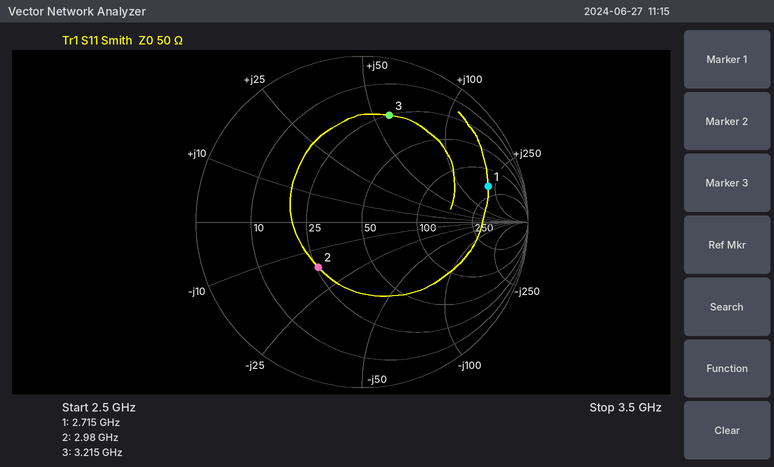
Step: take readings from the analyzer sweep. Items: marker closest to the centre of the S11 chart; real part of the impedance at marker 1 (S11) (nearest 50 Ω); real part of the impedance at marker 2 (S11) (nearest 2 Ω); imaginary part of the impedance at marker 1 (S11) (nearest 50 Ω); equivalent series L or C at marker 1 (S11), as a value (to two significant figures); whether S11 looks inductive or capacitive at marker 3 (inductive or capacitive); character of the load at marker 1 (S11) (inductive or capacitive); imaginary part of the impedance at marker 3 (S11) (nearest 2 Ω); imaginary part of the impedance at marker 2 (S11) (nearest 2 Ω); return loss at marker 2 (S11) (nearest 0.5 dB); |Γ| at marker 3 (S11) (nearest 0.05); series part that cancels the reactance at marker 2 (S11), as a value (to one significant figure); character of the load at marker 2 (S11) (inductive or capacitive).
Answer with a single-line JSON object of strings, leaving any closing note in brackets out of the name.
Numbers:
{"marker closest to the centre of the S11 chart": "marker 2", "real part of the impedance at marker 1 (S11)": "200 Ω", "real part of the impedance at marker 2 (S11)": "26 Ω", "imaginary part of the impedance at marker 1 (S11)": "+200 Ω", "equivalent series L or C at marker 1 (S11), as a value": "12 nH", "whether S11 looks inductive or capacitive at marker 3": "inductive", "character of the load at marker 1 (S11)": "inductive", "imaginary part of the impedance at marker 3 (S11)": "+58 Ω", "imaginary part of the impedance at marker 2 (S11)": "-16 Ω", "return loss at marker 2 (S11)": "8.5 dB", "|Γ| at marker 3 (S11)": "0.65", "series part that cancels the reactance at marker 2 (S11), as a value": "900 pH", "character of the load at marker 2 (S11)": "capacitive"}
